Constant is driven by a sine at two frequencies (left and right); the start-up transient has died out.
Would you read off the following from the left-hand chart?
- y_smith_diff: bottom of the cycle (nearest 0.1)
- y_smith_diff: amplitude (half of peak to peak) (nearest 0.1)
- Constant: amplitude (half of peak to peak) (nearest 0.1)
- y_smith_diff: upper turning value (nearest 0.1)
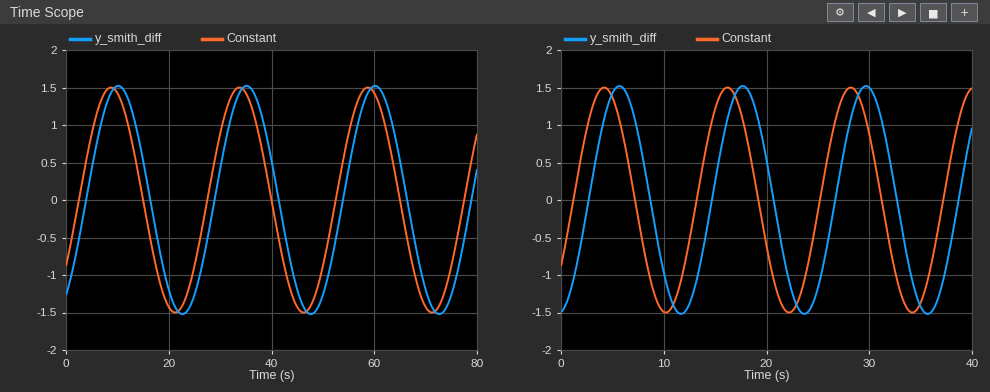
-1.5
1.5
1.5
1.5
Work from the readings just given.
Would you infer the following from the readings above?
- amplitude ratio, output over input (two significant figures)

1.0
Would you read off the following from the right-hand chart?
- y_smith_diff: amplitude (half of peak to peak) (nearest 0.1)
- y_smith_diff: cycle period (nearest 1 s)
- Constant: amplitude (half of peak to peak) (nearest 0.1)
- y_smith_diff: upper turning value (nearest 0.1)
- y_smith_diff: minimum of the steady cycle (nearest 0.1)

1.5
12 s
1.5
1.5
-1.5
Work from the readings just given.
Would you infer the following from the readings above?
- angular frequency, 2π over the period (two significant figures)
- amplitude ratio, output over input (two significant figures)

0.52 rad/s
1.0
